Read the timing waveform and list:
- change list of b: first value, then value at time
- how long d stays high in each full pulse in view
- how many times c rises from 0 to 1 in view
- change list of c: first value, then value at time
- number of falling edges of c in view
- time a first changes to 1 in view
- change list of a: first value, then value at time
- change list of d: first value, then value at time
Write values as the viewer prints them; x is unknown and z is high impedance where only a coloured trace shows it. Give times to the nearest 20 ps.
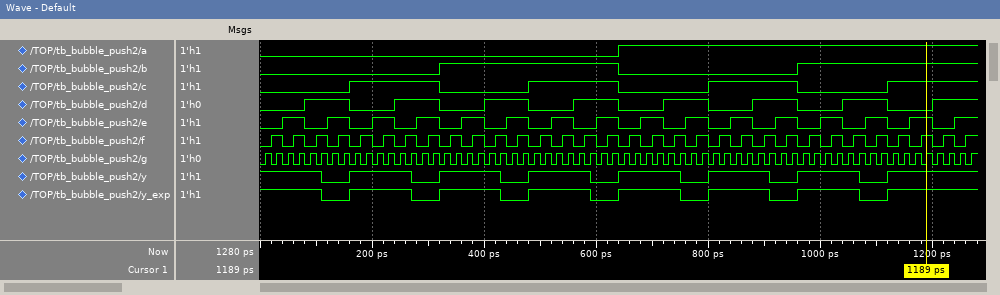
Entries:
0, 1 at 320 ps, 0 at 640 ps, 1 at 960 ps
80 ps, 80 ps, 80 ps, 80 ps, 80 ps, 80 ps, 80 ps
4
0, 1 at 160 ps, 0 at 320 ps, 1 at 480 ps, 0 at 640 ps, 1 at 800 ps, 0 at 960 ps, 1 at 1120 ps
3
640 ps
0, 1 at 640 ps
0, 1 at 80 ps, 0 at 160 ps, 1 at 240 ps, 0 at 320 ps, 1 at 400 ps, 0 at 480 ps, 1 at 560 ps, 0 at 640 ps, 1 at 720 ps, 0 at 800 ps, 1 at 880 ps, 0 at 960 ps, 1 at 1040 ps, 0 at 1120 ps, 1 at 1200 ps
